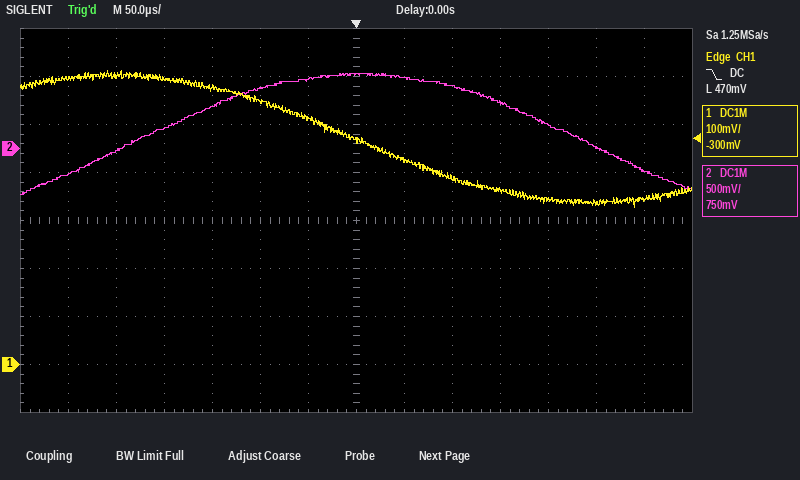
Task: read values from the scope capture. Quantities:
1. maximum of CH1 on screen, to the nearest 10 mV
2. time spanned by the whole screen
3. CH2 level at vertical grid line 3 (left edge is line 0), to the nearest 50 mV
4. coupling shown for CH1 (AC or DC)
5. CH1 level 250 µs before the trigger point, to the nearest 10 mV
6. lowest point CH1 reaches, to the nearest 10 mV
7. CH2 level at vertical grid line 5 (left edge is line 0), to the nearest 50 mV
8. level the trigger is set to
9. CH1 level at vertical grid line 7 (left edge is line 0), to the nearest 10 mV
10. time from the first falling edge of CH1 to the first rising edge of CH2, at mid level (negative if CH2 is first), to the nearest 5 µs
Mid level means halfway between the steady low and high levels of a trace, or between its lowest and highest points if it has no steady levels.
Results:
610 mV
700 µs
200 mV
DC
600 mV
330 mV
650 mV
470 mV
470 mV
-215 µs
